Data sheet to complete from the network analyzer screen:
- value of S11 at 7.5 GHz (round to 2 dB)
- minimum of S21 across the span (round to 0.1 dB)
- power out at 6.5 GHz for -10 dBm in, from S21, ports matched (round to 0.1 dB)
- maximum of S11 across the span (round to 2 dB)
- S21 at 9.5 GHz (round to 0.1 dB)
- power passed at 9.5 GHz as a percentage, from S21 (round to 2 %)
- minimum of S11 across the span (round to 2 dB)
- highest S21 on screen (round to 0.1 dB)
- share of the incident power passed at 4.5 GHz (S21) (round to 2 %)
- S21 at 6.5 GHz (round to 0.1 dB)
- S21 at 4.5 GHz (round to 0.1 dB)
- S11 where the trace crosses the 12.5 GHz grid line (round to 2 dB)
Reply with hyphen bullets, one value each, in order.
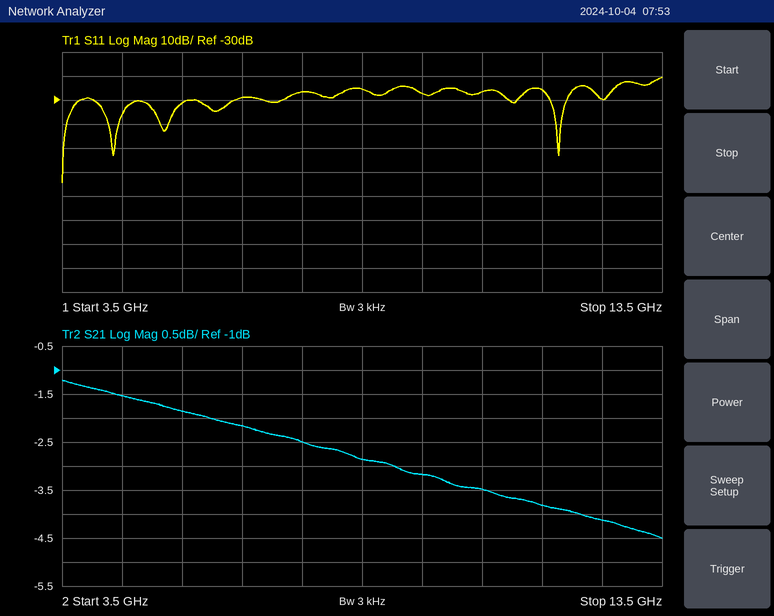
- -26 dB
- -4.5 dB
- -12.2 dBm
- -20 dB
- -3.2 dB
- 48 %
- -64 dB
- -1.2 dB
- 70 %
- -2.2 dB
- -1.5 dB
- -30 dB
